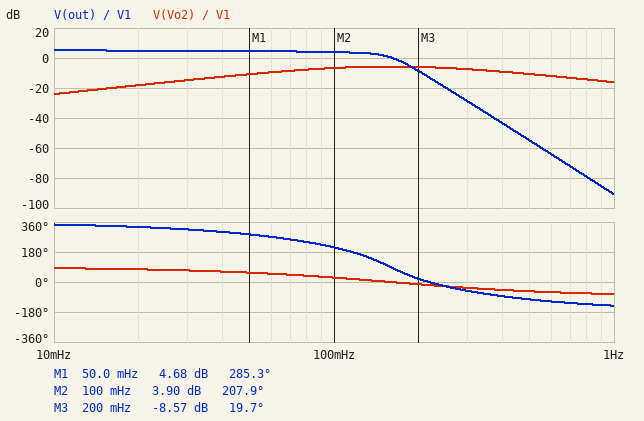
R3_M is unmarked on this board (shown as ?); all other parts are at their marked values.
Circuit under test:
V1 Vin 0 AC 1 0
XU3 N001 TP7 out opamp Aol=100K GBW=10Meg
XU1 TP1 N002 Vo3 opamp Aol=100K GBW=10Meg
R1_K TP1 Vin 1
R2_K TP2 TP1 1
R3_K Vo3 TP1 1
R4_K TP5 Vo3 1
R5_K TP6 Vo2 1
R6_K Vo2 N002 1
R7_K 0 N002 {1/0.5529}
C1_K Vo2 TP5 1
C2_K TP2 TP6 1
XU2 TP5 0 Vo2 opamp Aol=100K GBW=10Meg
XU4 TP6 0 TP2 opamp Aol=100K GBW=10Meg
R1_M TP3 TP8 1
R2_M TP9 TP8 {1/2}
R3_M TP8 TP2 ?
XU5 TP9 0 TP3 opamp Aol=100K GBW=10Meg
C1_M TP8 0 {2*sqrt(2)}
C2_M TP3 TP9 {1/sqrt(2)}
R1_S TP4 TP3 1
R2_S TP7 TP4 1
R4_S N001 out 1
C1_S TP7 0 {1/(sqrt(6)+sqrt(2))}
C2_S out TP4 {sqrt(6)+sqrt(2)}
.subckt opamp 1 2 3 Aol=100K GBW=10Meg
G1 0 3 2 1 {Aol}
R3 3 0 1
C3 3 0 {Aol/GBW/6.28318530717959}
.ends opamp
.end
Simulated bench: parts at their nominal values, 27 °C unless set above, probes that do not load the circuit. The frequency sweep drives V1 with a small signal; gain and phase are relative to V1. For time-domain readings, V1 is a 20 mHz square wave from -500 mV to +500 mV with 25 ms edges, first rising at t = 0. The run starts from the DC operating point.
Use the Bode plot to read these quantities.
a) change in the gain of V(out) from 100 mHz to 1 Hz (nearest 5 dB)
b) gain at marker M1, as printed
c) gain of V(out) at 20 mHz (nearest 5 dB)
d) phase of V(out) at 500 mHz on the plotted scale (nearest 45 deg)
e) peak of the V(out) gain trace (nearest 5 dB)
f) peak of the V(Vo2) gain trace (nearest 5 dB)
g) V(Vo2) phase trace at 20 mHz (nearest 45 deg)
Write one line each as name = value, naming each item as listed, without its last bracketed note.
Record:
change in the gain of V(out) from 100 mHz to 1 Hz = -95 dB
gain at marker M1, as printed = 4.68 dB
gain of V(out) at 20 mHz = 5 dB
phase of V(out) at 500 mHz on the plotted scale = -90 deg
peak of the V(out) gain trace = 5 dB
peak of the V(Vo2) gain trace = -5 dB
V(Vo2) phase trace at 20 mHz = 90 deg
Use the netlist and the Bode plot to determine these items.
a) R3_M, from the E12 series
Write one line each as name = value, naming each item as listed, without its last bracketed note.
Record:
R3_M, from the E12 series = 0.56 Ω
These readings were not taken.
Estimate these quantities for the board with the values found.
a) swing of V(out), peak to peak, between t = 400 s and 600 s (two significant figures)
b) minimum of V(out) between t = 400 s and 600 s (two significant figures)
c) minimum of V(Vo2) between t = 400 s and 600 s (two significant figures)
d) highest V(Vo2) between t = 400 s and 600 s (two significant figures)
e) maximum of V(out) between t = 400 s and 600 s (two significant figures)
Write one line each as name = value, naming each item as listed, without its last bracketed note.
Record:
swing of V(out), peak to peak, between t = 400 s and 600 s = 2.1 V
minimum of V(out) between t = 400 s and 600 s = -1.0 V
minimum of V(Vo2) between t = 400 s and 600 s = -380 mV
highest V(Vo2) between t = 400 s and 600 s = 380 mV
maximum of V(out) between t = 400 s and 600 s = 1.0 V
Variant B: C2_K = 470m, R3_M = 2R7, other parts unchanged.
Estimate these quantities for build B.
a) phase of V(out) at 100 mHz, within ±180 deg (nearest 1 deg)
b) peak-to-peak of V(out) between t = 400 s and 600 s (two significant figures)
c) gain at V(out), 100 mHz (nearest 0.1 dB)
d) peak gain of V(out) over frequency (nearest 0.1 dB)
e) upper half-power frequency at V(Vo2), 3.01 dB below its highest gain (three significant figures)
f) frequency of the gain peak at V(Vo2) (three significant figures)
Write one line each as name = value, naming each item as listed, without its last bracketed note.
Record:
phase of V(out) at 100 mHz, within ±180 deg = -114 deg
peak-to-peak of V(out) between t = 400 s and 600 s = 690 mV
gain at V(out), 100 mHz = -5.0 dB
peak gain of V(out) over frequency = -3.5 dB
upper half-power frequency at V(Vo2), 3.01 dB below its highest gain = 432 mHz
frequency of the gain peak at V(Vo2) = 232 mHz
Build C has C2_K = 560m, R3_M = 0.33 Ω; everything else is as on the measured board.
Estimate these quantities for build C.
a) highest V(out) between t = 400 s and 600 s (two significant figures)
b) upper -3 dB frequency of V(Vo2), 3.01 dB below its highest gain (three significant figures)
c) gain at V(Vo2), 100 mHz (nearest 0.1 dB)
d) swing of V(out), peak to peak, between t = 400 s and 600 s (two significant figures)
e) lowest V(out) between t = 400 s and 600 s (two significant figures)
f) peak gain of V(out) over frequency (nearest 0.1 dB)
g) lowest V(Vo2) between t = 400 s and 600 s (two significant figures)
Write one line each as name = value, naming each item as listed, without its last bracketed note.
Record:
highest V(out) between t = 400 s and 600 s = 1.9 V
upper -3 dB frequency of V(Vo2), 3.01 dB below its highest gain = 416 mHz
gain at V(Vo2), 100 mHz = -9.4 dB
swing of V(out), peak to peak, between t = 400 s and 600 s = 3.7 V
lowest V(out) between t = 400 s and 600 s = -1.9 V
peak gain of V(out) over frequency = 9.6 dB
lowest V(Vo2) between t = 400 s and 600 s = -340 mV
